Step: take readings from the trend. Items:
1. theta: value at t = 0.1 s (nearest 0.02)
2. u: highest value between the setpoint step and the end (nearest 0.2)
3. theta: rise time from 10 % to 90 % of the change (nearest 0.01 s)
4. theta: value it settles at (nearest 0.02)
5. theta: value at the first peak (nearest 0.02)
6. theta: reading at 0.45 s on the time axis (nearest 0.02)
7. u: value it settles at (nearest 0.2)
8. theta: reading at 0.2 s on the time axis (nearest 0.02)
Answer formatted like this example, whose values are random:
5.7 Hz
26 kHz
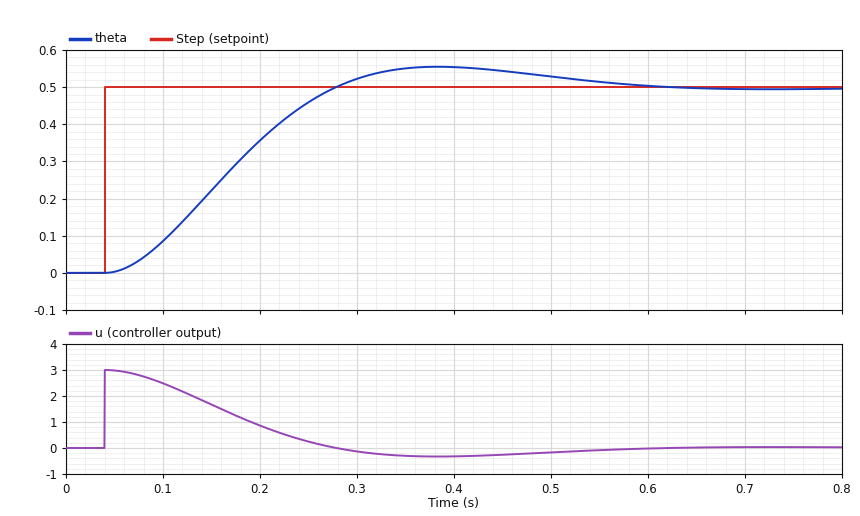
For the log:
0.08
3.0
0.16 s
0.50
0.56
0.54
0.0
0.36
